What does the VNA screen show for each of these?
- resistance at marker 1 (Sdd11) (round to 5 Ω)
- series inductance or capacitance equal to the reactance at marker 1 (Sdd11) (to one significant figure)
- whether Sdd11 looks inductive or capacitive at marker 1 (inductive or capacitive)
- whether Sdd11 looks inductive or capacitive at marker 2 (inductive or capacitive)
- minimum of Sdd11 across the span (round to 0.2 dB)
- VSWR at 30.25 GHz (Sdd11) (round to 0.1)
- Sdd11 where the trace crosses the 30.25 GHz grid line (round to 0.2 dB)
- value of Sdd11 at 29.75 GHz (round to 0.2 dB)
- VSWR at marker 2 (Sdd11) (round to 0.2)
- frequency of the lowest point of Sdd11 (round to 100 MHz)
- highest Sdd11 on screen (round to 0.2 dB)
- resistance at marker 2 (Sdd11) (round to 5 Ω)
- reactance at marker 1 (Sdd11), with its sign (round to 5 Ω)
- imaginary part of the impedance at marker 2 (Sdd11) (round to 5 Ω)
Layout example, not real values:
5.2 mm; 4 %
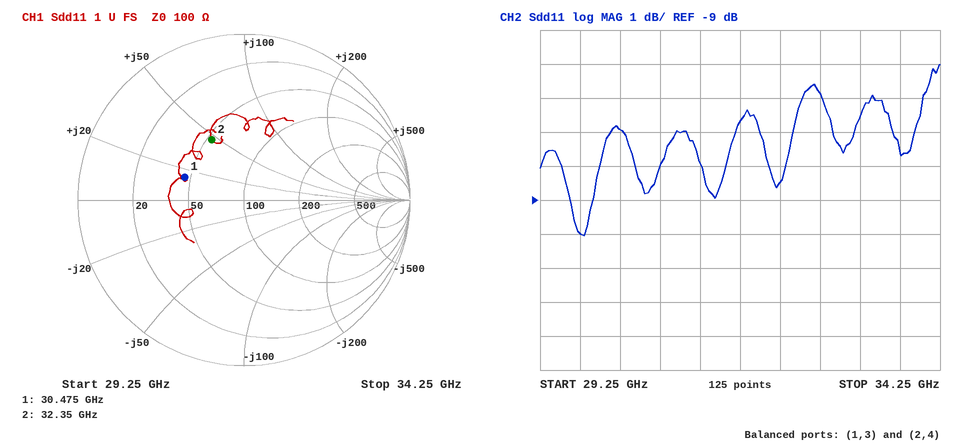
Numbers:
45 Ω; 80 pH; inductive; inductive; -10.0 dB; 2.6; -7.0 dB; -10.0 dB; 2.4; 29.8 GHz; -5.0 dB; 55 Ω; +15 Ω; +45 Ω
